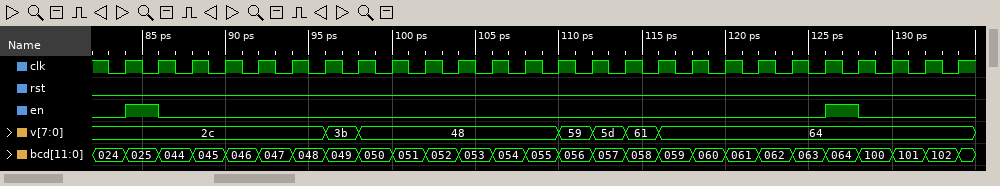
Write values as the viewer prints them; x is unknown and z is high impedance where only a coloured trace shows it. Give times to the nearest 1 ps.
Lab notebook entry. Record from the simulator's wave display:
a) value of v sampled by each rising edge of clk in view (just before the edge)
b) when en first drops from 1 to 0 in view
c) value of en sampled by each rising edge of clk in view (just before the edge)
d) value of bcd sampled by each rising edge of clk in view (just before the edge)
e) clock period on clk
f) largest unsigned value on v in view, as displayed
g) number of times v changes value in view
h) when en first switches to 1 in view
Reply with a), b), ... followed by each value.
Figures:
a) 2c, 2c, 2c, 2c, 2c, 2c, 2c, 3b, 48, 48, 48, 48, 48, 48, 59, 5d, 61, 64, 64, 64, 64, 64, 64, 64, 64, 64
b) 86 ps
c) 0 1 0 0 0 0 0 0 0 0 0 0 0 0 0 0 0 0 0 0 0 0 1 0 0 0
d) 024, 025, 044, 045, 046, 047, 048, 049, 050, 051, 052, 053, 054, 055, 056, 057, 058, 059, 060, 061, 062, 063, 064, 100, 101, 102
e) 2 ps
f) 64
g) 6
h) 84 ps
